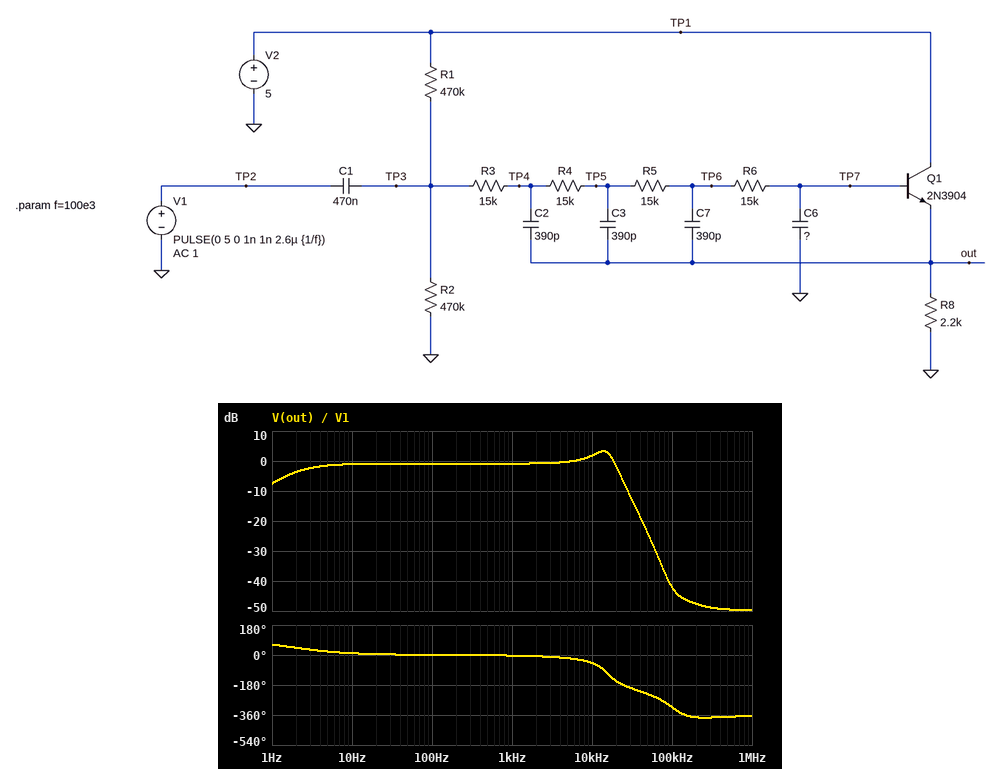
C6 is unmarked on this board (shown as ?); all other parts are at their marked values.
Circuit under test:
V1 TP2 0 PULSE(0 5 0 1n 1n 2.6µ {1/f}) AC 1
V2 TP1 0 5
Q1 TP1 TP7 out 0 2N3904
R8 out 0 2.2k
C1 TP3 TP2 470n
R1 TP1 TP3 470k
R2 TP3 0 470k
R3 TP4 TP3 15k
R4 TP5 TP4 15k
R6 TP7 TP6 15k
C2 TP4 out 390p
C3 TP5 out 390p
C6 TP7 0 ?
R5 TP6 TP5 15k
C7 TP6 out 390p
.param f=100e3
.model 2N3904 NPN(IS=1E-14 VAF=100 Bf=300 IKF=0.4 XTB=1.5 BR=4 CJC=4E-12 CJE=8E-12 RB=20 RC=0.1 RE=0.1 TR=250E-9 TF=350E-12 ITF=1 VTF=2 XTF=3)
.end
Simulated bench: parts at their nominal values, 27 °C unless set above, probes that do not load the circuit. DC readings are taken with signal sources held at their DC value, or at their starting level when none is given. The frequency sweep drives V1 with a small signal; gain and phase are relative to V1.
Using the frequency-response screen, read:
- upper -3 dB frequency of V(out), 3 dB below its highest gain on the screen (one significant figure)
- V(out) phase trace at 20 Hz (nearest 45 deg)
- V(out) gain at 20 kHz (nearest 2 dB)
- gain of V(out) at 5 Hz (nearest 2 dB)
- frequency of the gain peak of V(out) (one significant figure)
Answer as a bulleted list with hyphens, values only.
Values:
- 20 kHz
- 0 deg
- -2 dB
- -2 dB
- 10 kHz
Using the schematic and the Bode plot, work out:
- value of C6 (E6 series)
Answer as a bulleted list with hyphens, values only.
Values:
- 150 pF
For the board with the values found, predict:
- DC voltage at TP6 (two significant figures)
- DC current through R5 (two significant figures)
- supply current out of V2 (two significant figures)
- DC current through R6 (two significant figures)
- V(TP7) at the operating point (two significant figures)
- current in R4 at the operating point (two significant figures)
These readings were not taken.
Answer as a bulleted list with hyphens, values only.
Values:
- 2.0 V
- 1.9 µA
- 590 µA
- 1.9 µA
- 1.9 V
- 1.9 µA
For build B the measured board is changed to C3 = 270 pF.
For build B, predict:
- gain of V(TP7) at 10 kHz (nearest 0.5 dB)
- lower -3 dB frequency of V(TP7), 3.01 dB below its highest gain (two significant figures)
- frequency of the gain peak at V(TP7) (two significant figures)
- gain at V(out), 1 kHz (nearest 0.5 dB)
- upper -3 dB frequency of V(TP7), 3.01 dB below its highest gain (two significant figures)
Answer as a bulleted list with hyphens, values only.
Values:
- 1.5 dB
- 4.8 kHz
- 15 kHz
- -1.0 dB
- 20 kHz
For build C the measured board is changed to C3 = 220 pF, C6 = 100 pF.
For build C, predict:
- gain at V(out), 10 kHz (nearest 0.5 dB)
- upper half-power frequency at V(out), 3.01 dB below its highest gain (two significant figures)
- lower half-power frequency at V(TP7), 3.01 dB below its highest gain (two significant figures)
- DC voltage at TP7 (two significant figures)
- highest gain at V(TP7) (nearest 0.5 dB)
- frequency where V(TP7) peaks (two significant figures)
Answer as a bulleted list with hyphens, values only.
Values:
- 1.0 dB
- 24 kHz
- 12 kHz
- 1.9 V
- 5.0 dB
- 19 kHz
